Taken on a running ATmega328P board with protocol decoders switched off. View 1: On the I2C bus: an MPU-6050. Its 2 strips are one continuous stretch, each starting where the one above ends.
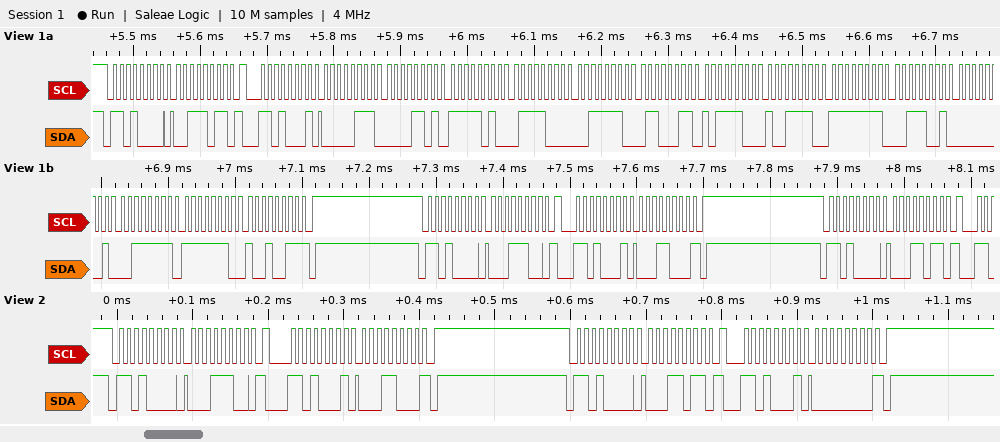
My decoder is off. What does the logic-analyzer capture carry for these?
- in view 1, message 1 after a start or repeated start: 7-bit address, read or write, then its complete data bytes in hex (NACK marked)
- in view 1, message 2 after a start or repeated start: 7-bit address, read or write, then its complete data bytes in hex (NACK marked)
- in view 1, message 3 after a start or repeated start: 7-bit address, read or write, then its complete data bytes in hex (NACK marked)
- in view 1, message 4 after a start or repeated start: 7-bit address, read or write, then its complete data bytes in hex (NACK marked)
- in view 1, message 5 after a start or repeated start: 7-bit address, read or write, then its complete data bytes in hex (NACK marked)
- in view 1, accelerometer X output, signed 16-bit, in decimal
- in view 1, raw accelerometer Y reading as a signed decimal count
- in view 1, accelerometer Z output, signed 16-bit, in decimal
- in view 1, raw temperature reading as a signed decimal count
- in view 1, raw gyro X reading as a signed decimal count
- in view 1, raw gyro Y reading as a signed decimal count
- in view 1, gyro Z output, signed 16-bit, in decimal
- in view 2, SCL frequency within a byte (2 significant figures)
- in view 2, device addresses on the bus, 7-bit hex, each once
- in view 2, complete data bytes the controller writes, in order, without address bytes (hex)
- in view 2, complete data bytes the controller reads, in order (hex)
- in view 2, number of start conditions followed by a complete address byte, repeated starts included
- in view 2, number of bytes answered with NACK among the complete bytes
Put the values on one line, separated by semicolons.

0x68 write: 3B; 0x68 read: 07 0D FA 78 3E 63 BC 9E FF 39 01 3F FE 93 NACK; 0x68 write: 1C; 0x68 read: 18 NACK; 0x68 write: 1B; 1805; -1416; 15971; -17250; -199; 319; -365; 100 kHz; 0x68; 1C 1B; 18 00; 4; 2
